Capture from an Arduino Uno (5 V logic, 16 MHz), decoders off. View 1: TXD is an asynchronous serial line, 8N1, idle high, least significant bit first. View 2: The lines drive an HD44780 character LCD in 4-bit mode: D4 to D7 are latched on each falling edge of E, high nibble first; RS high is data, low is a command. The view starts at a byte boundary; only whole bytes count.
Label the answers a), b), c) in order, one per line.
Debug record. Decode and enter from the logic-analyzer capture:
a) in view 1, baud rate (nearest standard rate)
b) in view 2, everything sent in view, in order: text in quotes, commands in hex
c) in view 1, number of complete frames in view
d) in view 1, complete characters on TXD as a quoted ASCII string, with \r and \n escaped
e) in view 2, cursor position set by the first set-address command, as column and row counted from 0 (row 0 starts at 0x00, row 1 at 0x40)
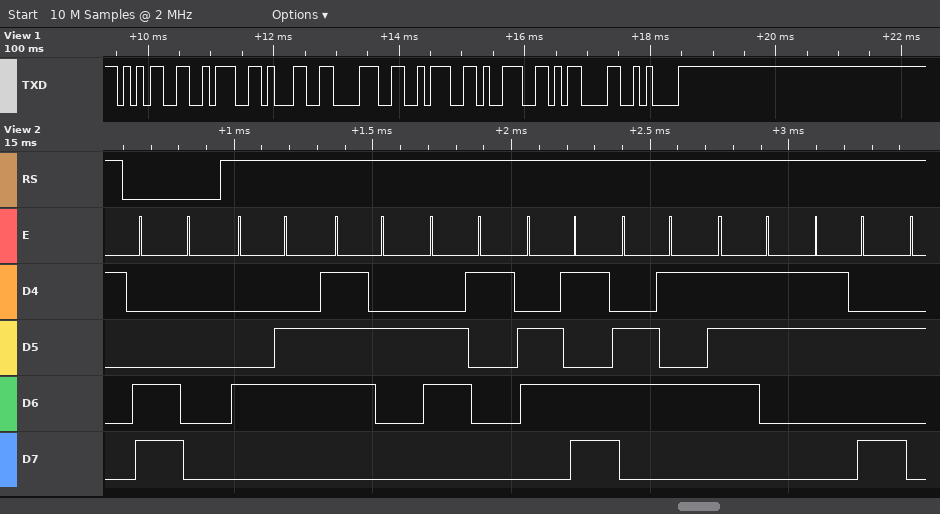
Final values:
a) 9600 baud
b) 0xC0 "Frames:"
c) 8
d) "5:18:9\r\n"
e) column 0, row 1
